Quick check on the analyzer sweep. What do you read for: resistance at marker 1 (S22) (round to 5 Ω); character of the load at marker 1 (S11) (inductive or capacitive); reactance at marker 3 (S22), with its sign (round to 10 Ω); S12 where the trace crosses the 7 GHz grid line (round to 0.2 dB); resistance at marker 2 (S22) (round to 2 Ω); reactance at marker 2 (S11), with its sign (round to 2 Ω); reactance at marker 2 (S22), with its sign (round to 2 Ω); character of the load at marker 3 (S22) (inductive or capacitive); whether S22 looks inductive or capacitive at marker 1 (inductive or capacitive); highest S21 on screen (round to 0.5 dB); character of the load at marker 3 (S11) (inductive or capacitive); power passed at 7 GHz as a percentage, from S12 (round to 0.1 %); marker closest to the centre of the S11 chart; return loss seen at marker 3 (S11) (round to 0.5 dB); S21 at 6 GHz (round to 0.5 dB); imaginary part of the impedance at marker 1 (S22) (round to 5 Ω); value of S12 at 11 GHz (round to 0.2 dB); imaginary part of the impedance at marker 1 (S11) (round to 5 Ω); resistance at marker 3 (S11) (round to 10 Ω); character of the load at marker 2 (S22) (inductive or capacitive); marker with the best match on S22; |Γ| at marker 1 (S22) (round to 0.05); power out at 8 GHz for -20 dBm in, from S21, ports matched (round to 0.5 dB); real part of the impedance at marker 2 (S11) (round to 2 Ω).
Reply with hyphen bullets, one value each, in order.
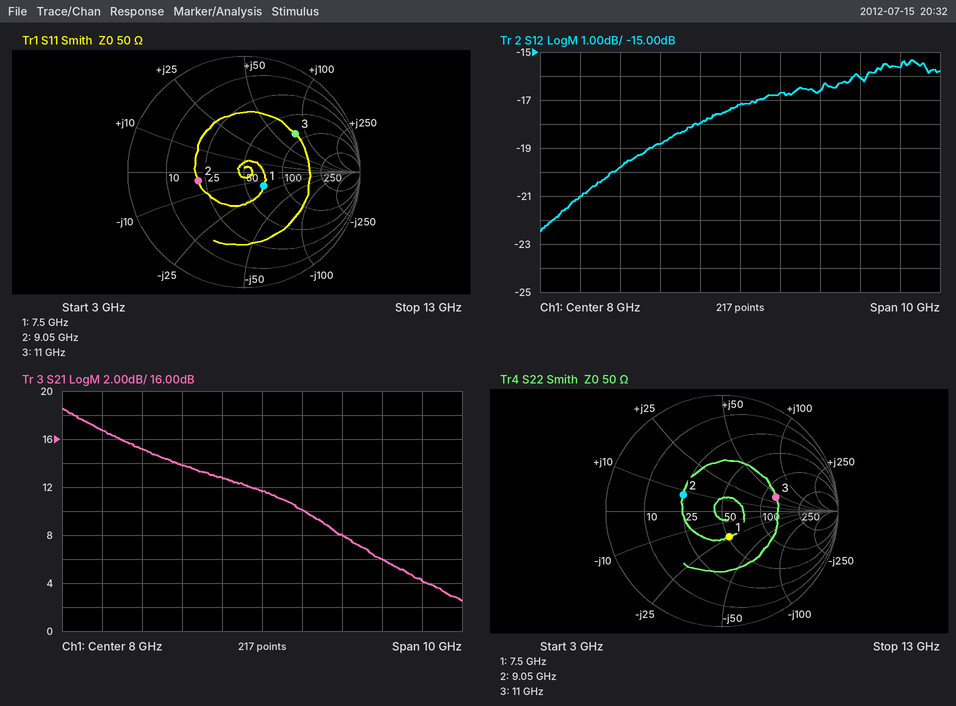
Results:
- 50 Ω
- capacitive
- +40 Ω
- -18.0 dB
- 24 Ω
- -4 Ω
- +8 Ω
- inductive
- capacitive
- 18.5 dB
- inductive
- 1.6 %
- marker 1
- 5.0 dB
- 14.0 dB
- -25 Ω
- -16.0 dB
- -15 Ω
- 80 Ω
- inductive
- marker 1
- 0.25
- -8.5 dBm
- 22 Ω
